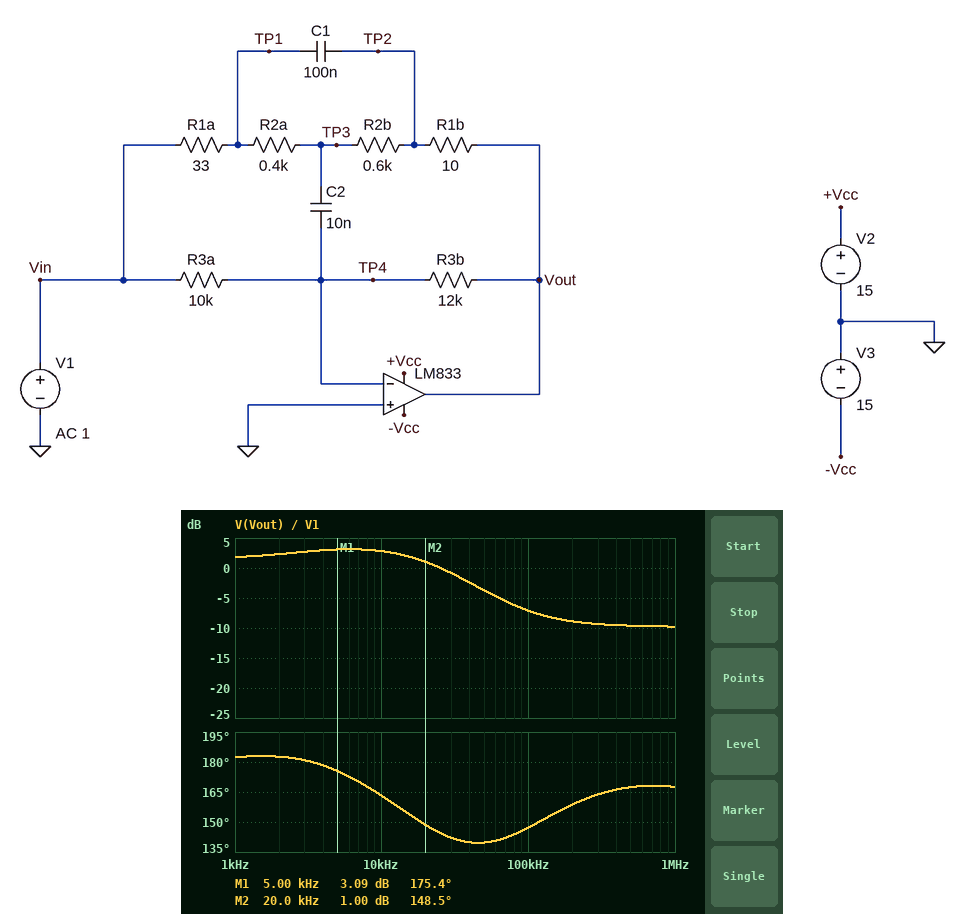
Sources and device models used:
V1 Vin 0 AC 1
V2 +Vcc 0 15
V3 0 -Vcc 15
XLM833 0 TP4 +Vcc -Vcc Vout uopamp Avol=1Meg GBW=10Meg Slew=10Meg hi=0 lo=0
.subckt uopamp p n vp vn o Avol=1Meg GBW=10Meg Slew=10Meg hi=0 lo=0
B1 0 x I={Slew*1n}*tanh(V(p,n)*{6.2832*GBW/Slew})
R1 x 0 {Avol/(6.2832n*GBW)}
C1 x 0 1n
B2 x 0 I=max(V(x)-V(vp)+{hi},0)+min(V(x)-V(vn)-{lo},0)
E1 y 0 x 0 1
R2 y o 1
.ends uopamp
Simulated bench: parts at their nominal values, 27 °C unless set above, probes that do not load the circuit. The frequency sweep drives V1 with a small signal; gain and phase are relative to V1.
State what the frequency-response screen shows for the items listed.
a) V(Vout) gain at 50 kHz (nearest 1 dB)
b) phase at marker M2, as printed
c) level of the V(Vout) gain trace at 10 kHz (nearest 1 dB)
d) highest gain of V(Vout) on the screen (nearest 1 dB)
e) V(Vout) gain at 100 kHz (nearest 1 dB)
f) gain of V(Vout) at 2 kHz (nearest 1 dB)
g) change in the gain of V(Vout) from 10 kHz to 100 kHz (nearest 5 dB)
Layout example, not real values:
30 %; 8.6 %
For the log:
-4 dB; 148.5 deg; 3 dB; 3 dB; -7 dB; 2 dB; -10 dB
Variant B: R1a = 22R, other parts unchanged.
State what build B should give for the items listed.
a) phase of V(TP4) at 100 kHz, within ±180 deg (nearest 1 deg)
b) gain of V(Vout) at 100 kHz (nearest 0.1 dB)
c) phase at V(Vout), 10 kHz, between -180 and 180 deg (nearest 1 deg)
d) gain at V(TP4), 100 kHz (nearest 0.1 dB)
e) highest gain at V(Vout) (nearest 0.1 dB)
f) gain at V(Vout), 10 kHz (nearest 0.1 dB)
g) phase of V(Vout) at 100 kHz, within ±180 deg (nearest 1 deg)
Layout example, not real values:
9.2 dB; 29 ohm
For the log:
65 deg; -4.0 dB; 171 deg; -43.6 dB; 3.2 dB; 3.1 dB; 152 deg
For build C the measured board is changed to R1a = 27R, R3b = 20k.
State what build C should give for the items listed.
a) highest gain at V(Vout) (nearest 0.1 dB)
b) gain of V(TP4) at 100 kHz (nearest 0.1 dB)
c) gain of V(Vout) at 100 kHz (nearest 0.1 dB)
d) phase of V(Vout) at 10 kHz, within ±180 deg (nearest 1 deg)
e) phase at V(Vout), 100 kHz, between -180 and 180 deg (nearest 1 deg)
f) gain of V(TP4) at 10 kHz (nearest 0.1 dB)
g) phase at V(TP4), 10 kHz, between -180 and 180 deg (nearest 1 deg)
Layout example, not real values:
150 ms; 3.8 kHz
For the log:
6.0 dB; -45.0 dB; -5.5 dB; 161 deg; 149 deg; -56.7 dB; 71 deg
